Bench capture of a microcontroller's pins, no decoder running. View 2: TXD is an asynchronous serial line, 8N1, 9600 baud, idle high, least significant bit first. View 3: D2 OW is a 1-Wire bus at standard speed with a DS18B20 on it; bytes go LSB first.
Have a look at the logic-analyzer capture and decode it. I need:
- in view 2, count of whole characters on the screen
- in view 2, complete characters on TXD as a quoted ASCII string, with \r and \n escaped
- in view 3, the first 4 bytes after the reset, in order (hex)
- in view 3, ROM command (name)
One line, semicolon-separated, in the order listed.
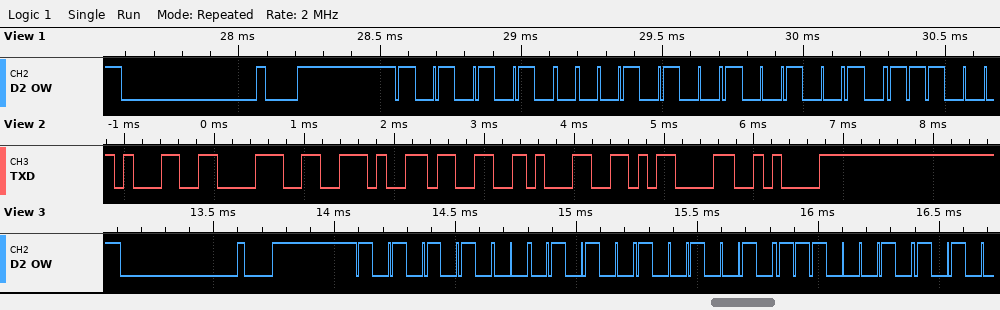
7; "18.31\r\n"; 55 28 49 47; Match ROM
